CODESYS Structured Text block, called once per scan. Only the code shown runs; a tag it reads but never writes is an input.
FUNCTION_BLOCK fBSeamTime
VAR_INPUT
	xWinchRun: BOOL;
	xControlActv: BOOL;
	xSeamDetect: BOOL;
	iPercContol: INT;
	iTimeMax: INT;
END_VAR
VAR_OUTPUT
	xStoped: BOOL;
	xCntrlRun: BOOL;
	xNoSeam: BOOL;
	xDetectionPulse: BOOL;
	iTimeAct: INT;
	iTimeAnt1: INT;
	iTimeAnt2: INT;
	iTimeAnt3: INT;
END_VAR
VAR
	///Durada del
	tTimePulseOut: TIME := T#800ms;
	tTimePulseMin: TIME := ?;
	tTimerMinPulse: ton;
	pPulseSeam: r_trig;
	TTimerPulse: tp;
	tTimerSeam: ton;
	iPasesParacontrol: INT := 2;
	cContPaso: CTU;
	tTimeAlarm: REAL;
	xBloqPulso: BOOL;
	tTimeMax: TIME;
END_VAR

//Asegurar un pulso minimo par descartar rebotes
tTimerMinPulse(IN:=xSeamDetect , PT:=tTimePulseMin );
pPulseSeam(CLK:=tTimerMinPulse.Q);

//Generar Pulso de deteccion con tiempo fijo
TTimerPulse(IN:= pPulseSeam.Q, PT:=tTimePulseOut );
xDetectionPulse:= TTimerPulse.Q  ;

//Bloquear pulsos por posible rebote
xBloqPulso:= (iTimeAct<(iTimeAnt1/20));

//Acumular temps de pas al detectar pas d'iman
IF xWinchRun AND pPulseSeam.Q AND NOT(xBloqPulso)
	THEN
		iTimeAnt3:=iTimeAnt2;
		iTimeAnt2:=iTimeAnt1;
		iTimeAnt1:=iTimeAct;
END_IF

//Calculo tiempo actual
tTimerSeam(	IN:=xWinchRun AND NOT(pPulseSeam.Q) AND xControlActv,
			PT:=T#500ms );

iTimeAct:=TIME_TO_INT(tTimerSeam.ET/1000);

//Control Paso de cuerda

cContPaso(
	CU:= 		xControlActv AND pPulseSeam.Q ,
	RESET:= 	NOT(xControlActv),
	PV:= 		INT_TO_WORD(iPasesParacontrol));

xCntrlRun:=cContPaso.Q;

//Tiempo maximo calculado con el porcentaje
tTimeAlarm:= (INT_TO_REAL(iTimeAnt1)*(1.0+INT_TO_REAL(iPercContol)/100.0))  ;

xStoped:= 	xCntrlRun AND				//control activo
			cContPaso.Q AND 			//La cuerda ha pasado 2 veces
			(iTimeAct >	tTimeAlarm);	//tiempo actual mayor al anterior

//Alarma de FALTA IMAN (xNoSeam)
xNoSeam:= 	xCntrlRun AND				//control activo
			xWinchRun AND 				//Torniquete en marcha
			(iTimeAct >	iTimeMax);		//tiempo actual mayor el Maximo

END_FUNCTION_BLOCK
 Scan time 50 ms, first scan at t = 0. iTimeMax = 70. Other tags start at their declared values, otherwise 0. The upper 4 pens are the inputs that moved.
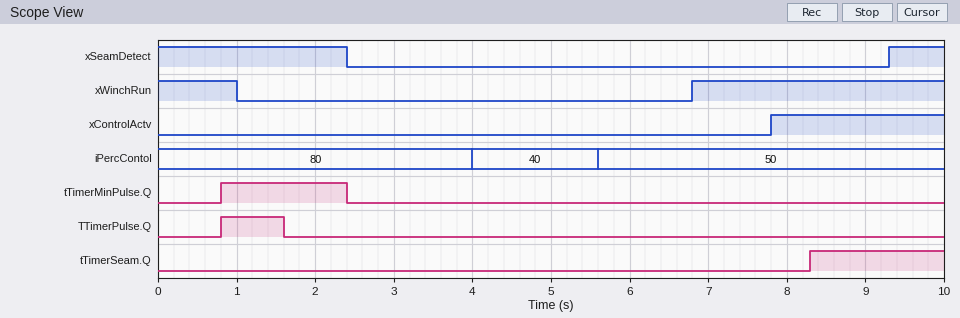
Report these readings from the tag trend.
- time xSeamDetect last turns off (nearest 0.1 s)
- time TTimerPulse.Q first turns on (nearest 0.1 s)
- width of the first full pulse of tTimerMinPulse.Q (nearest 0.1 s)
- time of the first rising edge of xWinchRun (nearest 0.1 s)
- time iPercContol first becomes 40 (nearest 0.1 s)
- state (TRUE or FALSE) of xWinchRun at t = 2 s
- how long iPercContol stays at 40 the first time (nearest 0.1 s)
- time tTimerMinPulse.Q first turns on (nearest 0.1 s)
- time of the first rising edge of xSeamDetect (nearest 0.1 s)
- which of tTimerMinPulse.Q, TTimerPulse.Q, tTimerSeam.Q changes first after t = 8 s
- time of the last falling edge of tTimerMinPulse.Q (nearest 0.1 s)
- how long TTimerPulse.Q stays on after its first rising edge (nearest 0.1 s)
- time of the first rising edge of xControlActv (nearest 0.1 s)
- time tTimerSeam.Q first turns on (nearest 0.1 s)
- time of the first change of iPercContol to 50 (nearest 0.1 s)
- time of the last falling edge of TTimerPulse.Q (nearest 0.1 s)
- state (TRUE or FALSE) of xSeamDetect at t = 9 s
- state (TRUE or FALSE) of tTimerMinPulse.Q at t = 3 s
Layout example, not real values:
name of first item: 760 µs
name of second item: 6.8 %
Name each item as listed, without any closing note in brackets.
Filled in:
time xSeamDetect last turns off: 2.4 s
time TTimerPulse.Q first turns on: 0.8 s
width of the first full pulse of tTimerMinPulse.Q: 1.6 s
time of the first rising edge of xWinchRun: 6.8 s
time iPercContol first becomes 40: 4.0 s
state (TRUE or FALSE) of xWinchRun at t = 2 s: FALSE
how long iPercContol stays at 40 the first time: 1.6 s
time tTimerMinPulse.Q first turns on: 0.8 s
time of the first rising edge of xSeamDetect: 9.3 s
which of tTimerMinPulse.Q, TTimerPulse.Q, tTimerSeam.Q changes first after t = 8 s: tTimerSeam.Q
time of the last falling edge of tTimerMinPulse.Q: 2.4 s
how long TTimerPulse.Q stays on after its first rising edge: 0.8 s
time of the first rising edge of xControlActv: 7.8 s
time tTimerSeam.Q first turns on: 8.3 s
time of the first change of iPercContol to 50: 5.6 s
time of the last falling edge of TTimerPulse.Q: 1.6 s
state (TRUE or FALSE) of xSeamDetect at t = 9 s: FALSE
state (TRUE or FALSE) of tTimerMinPulse.Q at t = 3 s: FALSE
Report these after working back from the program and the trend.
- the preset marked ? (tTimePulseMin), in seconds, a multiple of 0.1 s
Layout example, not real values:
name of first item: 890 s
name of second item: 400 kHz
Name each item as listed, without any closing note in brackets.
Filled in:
the preset marked ? (tTimePulseMin), in seconds, a multiple of 0.1 s: 0.8 s
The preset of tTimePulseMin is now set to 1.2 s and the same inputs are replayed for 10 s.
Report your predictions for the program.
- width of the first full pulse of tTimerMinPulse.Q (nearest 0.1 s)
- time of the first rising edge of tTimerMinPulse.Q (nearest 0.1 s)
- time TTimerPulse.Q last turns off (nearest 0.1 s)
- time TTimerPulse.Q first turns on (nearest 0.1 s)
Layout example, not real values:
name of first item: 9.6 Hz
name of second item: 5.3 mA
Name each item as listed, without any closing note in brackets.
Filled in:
width of the first full pulse of tTimerMinPulse.Q: 1.2 s
time of the first rising edge of tTimerMinPulse.Q: 1.2 s
time TTimerPulse.Q last turns off: 2.0 s
time TTimerPulse.Q first turns on: 1.2 s
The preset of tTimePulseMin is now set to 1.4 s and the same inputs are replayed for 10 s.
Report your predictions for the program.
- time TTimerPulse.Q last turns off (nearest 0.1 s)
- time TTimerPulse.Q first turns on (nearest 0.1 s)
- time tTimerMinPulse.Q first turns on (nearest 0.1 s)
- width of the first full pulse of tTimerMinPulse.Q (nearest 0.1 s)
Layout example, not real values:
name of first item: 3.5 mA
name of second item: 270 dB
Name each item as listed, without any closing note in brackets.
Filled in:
time TTimerPulse.Q last turns off: 2.2 s
time TTimerPulse.Q first turns on: 1.4 s
time tTimerMinPulse.Q first turns on: 1.4 s
width of the first full pulse of tTimerMinPulse.Q: 1.0 s
